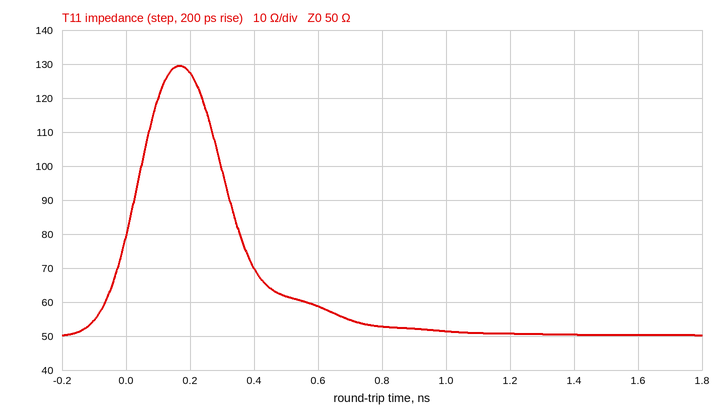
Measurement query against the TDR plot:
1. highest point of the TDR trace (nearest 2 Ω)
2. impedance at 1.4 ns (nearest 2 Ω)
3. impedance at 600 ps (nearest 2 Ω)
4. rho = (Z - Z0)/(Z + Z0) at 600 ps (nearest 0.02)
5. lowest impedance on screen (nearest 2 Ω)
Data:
130 Ω
50 Ω
58 Ω
+0.08
50 Ω
